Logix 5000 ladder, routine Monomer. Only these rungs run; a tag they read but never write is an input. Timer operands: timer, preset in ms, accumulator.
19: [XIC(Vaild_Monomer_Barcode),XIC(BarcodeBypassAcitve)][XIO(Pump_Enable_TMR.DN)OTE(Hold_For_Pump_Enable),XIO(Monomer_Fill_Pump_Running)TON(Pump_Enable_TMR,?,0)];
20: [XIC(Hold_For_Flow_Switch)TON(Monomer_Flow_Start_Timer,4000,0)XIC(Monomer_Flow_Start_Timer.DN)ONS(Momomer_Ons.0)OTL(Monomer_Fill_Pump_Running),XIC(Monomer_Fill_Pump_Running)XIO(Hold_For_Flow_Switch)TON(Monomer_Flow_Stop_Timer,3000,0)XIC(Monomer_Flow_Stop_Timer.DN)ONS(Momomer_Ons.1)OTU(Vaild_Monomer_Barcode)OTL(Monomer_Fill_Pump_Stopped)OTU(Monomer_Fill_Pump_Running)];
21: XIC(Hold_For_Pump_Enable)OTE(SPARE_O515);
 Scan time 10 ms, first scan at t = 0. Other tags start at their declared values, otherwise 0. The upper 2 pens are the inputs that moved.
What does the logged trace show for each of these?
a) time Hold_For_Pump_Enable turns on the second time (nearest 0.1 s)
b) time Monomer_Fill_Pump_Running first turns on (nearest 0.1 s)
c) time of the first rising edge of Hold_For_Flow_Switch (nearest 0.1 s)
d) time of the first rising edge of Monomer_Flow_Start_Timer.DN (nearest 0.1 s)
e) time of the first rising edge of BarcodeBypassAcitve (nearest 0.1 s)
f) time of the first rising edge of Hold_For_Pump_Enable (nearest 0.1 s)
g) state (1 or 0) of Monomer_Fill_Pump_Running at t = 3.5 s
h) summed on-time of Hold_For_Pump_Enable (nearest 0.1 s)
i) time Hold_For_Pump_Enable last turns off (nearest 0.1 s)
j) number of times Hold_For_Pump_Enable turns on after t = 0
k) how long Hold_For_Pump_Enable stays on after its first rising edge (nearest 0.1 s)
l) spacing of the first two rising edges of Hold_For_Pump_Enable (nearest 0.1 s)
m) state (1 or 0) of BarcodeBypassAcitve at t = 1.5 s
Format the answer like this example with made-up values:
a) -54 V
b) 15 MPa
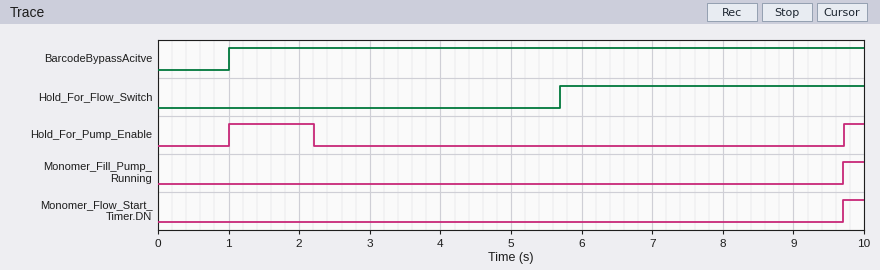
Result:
a) 9.7 s
b) 9.7 s
c) 5.7 s
d) 9.7 s
e) 1.0 s
f) 1.0 s
g) 0
h) 1.5 s
i) 2.2 s
j) 2
k) 1.2 s
l) 8.7 s
m) 1
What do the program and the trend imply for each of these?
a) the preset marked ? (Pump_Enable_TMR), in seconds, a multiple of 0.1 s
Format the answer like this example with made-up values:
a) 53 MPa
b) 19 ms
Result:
a) 1.2 s
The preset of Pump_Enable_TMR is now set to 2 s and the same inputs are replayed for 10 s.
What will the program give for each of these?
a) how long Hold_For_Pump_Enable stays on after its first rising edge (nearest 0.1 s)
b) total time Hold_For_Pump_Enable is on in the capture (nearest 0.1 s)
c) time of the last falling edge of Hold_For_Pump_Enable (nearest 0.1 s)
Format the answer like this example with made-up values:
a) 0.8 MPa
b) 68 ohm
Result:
a) 2.0 s
b) 2.3 s
c) 3.0 s
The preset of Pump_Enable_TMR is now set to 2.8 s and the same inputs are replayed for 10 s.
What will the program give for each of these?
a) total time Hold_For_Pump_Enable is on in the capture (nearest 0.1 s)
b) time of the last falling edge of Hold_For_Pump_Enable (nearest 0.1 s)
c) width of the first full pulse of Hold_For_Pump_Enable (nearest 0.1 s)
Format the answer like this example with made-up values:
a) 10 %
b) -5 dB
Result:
a) 3.1 s
b) 3.8 s
c) 2.8 s
